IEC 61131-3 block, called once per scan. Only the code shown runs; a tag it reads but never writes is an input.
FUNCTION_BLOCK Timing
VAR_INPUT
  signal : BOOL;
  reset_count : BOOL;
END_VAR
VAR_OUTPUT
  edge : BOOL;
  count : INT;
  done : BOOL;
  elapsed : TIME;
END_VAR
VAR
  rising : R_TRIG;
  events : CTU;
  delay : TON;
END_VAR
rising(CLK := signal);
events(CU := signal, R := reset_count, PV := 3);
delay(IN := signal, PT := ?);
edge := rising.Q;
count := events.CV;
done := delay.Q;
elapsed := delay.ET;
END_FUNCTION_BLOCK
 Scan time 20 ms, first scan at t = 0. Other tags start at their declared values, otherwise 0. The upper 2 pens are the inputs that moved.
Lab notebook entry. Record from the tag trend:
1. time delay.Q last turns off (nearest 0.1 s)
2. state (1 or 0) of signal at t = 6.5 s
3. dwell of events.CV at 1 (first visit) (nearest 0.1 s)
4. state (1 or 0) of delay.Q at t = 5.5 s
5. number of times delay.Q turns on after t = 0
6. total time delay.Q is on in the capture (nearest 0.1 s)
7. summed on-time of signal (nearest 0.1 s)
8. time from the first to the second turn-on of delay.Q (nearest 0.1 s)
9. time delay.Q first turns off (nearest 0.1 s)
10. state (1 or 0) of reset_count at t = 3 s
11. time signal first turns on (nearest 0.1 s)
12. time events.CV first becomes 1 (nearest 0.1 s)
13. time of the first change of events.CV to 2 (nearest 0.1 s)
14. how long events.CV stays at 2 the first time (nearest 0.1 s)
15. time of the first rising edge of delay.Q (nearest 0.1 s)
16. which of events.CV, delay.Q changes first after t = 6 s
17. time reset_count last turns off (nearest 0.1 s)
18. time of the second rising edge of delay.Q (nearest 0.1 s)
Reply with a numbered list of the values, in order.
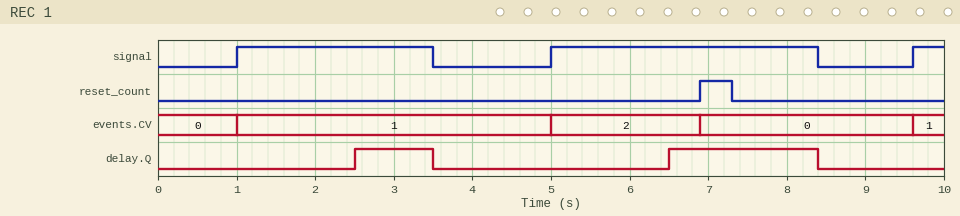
1. 8.4 s
2. 1
3. 4.0 s
4. 0
5. 2
6. 2.9 s
7. 6.3 s
8. 4.0 s
9. 3.5 s
10. 0
11. 1.0 s
12. 1.0 s
13. 5.0 s
14. 1.9 s
15. 2.5 s
16. delay.Q
17. 7.3 s
18. 6.5 s
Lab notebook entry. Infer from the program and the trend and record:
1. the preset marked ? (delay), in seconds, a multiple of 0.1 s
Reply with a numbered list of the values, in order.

1. 1.5 s
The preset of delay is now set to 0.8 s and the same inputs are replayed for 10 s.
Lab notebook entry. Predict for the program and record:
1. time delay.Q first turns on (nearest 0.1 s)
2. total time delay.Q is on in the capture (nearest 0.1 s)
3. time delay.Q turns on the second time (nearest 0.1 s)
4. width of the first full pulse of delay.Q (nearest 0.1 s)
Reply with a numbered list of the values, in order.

1. 1.8 s
2. 4.3 s
3. 5.8 s
4. 1.7 s
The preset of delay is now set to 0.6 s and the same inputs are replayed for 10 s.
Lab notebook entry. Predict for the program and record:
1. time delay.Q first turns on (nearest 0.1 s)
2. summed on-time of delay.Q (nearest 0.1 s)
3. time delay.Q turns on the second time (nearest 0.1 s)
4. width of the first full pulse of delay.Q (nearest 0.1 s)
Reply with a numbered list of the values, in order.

1. 1.6 s
2. 4.7 s
3. 5.6 s
4. 1.9 s
